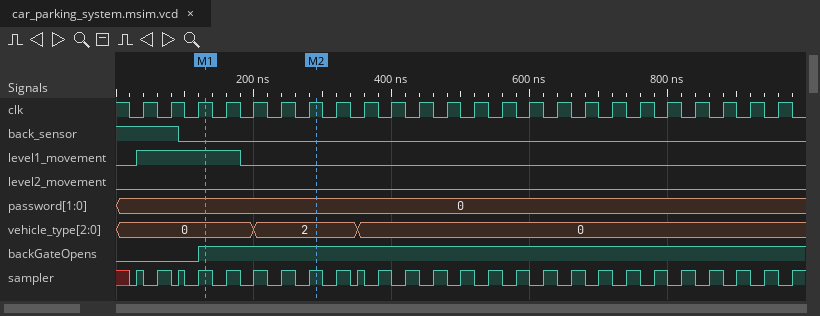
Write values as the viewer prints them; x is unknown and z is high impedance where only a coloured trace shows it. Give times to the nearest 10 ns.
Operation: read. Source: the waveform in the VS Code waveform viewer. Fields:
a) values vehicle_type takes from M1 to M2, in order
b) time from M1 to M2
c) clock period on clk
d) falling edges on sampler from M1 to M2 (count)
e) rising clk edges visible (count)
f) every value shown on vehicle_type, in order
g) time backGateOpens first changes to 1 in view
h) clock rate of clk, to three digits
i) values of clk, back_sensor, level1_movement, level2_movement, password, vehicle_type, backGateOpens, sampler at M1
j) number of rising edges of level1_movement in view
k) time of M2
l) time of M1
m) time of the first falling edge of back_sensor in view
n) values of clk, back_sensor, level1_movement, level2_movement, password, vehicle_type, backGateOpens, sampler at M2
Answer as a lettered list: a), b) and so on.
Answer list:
a) 0, 2
b) 160 ns
c) 40 ns
d) 4
e) 24
f) 0, 2, 0
g) 120 ns
h) 25.0 MHz
i) clk=1, back_sensor=0, level1_movement=1, level2_movement=0, password=0, vehicle_type=0, backGateOpens=1, sampler=1
j) 1
k) 290 ns
l) 130 ns
m) 90 ns
n) clk=1, back_sensor=0, level1_movement=0, level2_movement=0, password=0, vehicle_type=2, backGateOpens=1, sampler=1
